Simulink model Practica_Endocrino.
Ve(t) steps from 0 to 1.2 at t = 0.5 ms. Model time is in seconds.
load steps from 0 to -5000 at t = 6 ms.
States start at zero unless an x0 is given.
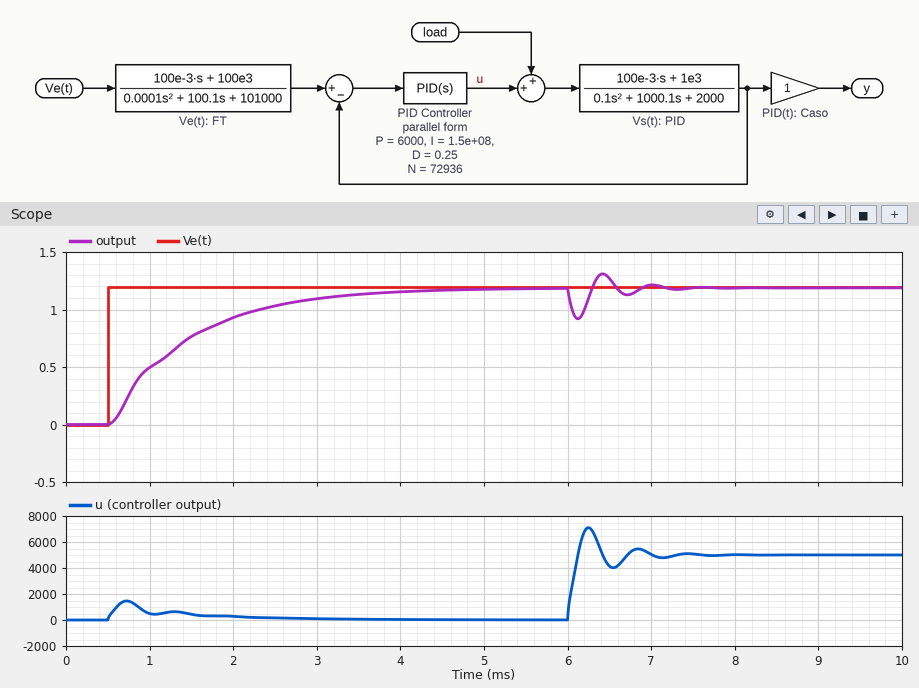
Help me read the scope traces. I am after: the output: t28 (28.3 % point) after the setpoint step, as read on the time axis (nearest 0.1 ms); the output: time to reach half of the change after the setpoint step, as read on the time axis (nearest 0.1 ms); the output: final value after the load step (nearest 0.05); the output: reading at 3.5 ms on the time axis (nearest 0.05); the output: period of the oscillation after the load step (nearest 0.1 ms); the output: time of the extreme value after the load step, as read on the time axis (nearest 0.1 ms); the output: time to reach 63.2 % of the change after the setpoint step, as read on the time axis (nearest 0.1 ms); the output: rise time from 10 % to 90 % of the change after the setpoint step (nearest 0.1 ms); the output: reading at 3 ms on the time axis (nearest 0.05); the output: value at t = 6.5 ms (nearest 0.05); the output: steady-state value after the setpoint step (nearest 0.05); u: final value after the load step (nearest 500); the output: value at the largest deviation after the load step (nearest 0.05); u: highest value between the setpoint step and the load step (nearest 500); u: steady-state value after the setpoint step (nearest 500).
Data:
0.8 ms
1.2 ms
1.20
1.15
0.6 ms
6.1 ms
1.5 ms
2.1 ms
1.10
1.25
1.20
5000
0.90
1500
0
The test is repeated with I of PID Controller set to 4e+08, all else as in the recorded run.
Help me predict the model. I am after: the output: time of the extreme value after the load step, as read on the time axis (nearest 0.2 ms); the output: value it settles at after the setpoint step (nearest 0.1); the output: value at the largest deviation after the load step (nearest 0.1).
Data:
6.0 ms
1.2
1.0
